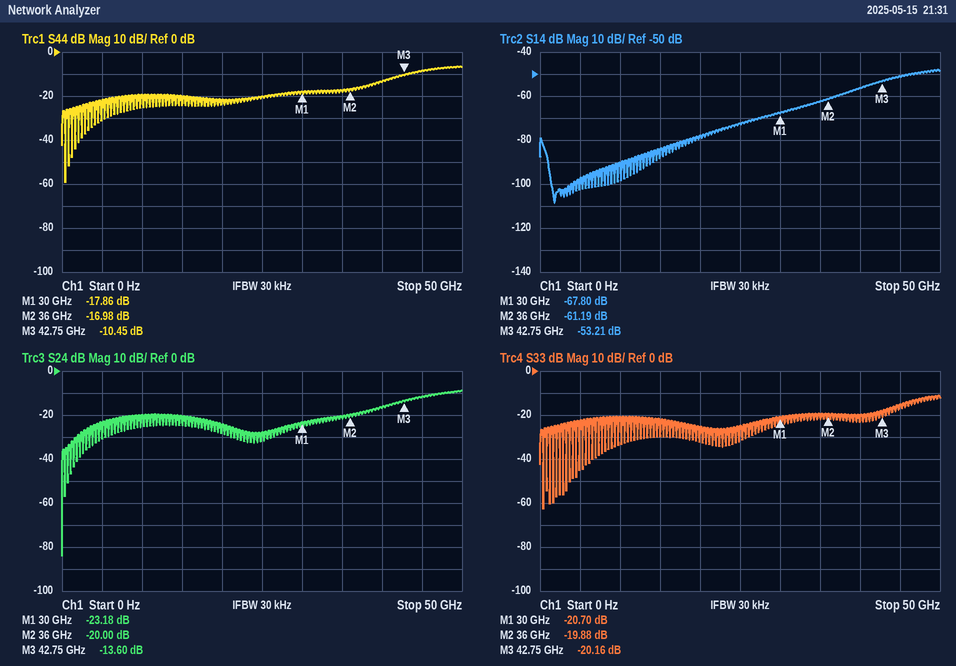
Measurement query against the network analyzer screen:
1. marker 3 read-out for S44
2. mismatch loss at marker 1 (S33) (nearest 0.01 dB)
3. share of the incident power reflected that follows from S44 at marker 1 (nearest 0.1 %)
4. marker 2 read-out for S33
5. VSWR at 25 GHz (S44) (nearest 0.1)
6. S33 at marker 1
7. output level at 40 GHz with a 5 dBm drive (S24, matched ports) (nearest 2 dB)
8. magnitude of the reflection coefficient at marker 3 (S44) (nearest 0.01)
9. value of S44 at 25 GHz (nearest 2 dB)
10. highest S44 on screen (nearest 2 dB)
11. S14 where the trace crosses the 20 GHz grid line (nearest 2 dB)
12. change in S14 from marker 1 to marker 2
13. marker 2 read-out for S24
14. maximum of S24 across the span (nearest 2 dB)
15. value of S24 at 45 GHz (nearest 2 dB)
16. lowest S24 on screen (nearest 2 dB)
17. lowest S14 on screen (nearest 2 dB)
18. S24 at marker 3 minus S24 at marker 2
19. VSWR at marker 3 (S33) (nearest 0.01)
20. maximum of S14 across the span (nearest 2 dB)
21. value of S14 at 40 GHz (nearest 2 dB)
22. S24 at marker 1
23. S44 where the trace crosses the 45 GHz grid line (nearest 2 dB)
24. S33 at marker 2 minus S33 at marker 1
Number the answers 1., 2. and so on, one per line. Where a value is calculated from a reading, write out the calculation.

1. -10.45 dB
2. −10 log10(1 − 10^(-20.7/10)) ≈ 0.04 dB
3. 10^(-17.86/10) ≈ 1.6 %
4. -19.88 dB
5. |Γ| = 10^(-20/20) = 0.1000; VSWR = (1 + 0.1000)/(1 − 0.1000) ≈ 1.2
6. -20.70 dB
7. 5 dBm + (-16 dB) = -12 dBm
8. 10^(-10.45/20) ≈ 0.30
9. -20 dB
10. -6 dB
11. -78 dB
12. -61.19 − (-67.8) = 6.61 dB
13. -20.00 dB
14. -8 dB
15. -12 dB
16. -84 dB
17. -108 dB
18. -13.6 − (-20) = 6.40 dB
19. (1 + 0.0982)/(1 − 0.0982) ≈ 1.22
20. -48 dB
21. -56 dB
22. -23.18 dB
23. -8 dB
24. -19.88 − (-20.7) = 0.82 dB
